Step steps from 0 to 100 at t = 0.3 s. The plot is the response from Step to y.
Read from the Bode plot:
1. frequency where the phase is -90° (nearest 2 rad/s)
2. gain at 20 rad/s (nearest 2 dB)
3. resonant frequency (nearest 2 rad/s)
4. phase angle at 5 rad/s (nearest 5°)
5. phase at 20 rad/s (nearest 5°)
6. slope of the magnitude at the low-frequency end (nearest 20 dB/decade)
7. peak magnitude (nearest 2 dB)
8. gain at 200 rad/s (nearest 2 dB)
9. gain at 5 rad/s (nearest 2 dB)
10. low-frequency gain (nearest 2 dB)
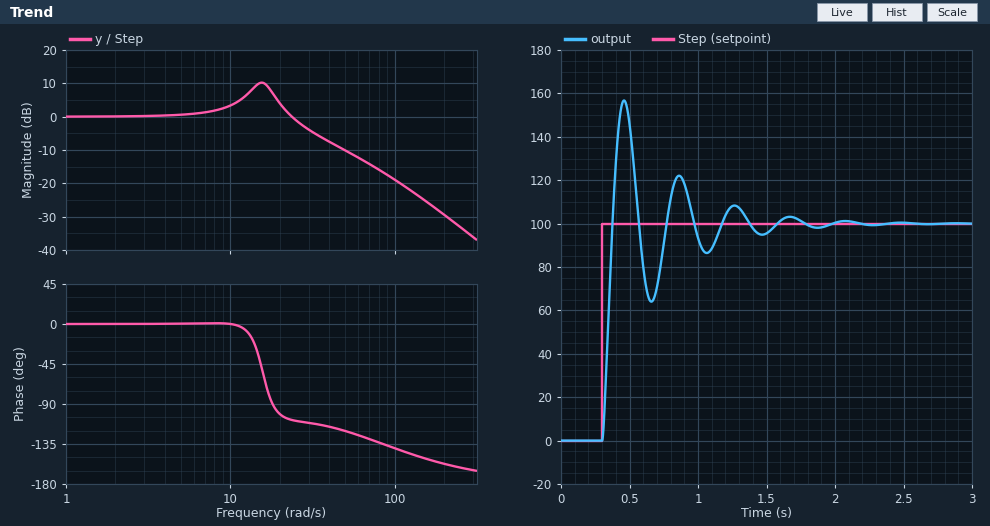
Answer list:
18 rad/s
4 dB
16 rad/s
0°
-100°
0 dB/decade
10 dB
-30 dB
0 dB
0 dB
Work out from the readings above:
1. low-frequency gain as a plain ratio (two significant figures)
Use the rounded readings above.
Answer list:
1.0
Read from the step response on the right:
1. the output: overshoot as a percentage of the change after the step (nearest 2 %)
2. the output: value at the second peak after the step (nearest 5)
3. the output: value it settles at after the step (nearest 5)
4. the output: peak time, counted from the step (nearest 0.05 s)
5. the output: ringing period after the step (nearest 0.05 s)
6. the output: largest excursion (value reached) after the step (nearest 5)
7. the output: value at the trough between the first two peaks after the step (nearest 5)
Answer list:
56 %
120
100
0.15 s
0.40 s
155
65
